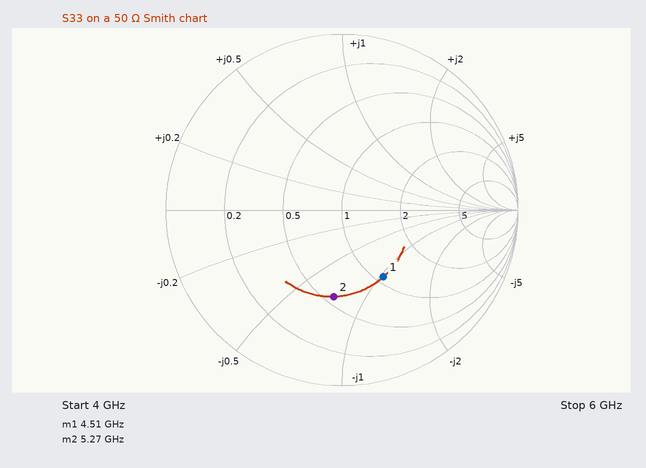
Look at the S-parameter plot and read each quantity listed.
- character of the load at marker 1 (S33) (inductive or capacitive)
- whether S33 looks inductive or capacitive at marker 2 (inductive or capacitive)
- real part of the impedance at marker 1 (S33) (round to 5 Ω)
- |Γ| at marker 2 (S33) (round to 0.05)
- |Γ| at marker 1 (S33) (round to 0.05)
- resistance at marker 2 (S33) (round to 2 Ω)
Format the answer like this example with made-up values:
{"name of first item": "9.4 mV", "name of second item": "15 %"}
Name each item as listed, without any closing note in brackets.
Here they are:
{"character of the load at marker 1 (S33)": "capacitive", "whether S33 looks inductive or capacitive at marker 2": "capacitive", "real part of the impedance at marker 1 (S33)": "55 Ω", "|Γ| at marker 2 (S33)": "0.50", "|Γ| at marker 1 (S33)": "0.45", "resistance at marker 2 (S33)": "28 Ω"}
